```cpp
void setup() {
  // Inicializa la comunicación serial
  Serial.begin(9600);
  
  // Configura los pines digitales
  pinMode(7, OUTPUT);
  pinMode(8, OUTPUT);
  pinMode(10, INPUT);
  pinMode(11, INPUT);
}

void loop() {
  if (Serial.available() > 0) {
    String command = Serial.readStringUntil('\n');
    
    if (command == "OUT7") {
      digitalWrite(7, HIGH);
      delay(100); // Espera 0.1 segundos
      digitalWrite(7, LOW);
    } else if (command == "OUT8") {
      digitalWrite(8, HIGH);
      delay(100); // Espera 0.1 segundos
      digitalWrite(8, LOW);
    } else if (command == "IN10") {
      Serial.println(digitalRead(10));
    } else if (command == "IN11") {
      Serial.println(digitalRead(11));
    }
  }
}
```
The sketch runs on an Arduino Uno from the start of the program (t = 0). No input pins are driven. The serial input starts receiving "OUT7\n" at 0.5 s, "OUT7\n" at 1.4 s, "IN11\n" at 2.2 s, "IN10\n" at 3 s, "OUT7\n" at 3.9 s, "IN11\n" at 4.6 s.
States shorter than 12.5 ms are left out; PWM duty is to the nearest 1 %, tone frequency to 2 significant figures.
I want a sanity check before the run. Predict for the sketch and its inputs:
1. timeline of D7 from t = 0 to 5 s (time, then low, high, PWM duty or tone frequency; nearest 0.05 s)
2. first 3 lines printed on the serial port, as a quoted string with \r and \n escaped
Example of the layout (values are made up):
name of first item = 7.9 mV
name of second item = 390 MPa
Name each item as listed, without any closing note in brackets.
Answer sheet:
timeline of D7 from t = 0 to 5 s = 0 s low; 0.5 s high; 0.6 s low; 1.4 s high; 1.5 s low; 3.9 s high; 4 s low
first 3 lines printed on the serial port, as a quoted string with \r and \n escaped = "0\r\n0\r\n0\r\n"
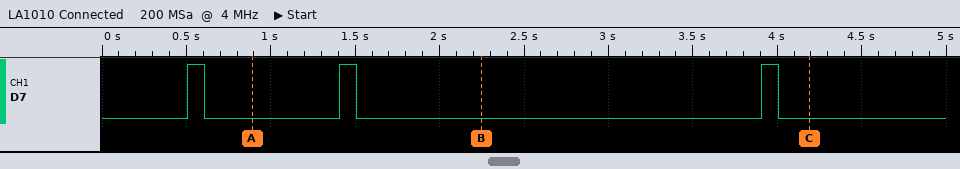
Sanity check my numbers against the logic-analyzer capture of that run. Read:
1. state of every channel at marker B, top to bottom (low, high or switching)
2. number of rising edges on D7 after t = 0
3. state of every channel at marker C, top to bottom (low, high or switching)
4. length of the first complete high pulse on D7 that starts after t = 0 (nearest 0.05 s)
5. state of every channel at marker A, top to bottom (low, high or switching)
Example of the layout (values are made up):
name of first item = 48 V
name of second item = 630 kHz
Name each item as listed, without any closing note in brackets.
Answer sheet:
state of every channel at marker B, top to bottom = D7 low
number of rising edges on D7 after t = 0 = 3
state of every channel at marker C, top to bottom = D7 low
length of the first complete high pulse on D7 that starts after t = 0 = 0.10 s
state of every channel at marker A, top to bottom = D7 low
